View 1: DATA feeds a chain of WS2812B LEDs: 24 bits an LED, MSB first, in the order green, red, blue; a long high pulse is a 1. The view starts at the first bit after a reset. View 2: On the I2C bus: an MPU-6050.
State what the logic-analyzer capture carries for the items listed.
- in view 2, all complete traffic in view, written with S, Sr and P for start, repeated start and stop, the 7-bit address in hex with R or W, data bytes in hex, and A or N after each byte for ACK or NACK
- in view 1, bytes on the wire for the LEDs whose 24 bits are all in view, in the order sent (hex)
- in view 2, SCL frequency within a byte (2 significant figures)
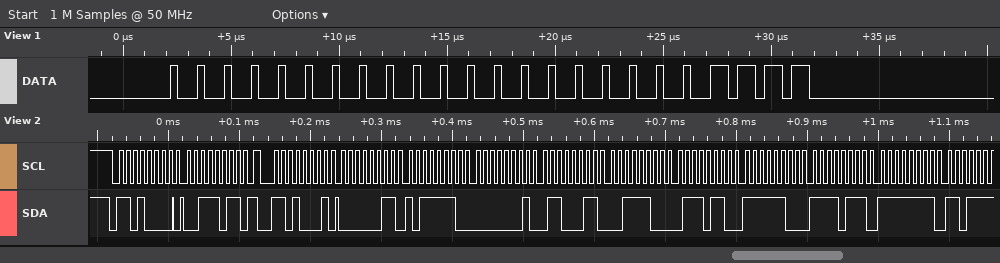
S 68W A 3B A Sr 68R A 03 A BE A 01 A 63 A 3C A 76 A FC A F7 A FF A
00 00 0F
100 kHz
